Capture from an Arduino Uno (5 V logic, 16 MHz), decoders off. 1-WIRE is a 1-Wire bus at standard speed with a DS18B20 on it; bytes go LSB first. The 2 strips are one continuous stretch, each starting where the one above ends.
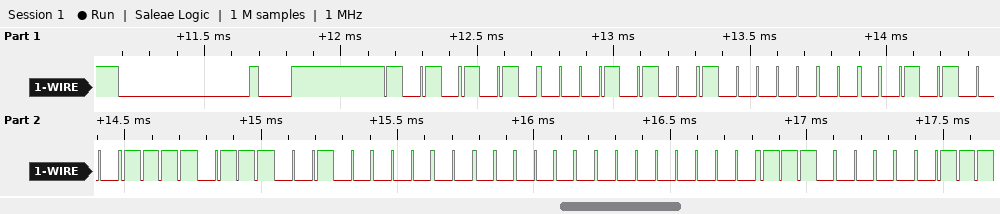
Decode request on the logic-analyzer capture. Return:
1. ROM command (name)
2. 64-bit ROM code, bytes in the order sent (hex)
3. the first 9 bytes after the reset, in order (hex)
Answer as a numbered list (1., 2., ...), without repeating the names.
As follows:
1. Match ROM
2. 28 01 14 EF 04 00 00 07
3. 55 28 01 14 EF 04 00 00 07
